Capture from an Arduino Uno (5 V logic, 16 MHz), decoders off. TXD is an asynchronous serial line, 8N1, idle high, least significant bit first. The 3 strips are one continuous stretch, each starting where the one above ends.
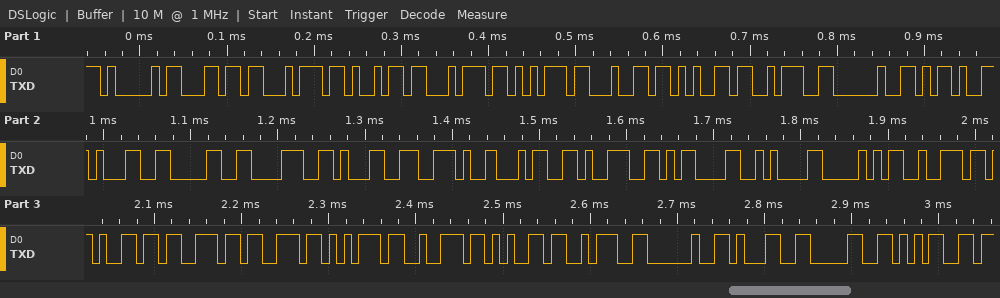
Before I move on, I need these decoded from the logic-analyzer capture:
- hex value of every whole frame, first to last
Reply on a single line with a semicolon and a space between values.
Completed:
41 6C 74 69 74 75 64 65 3A 20 2D 31 30 38 31 2E 34 39 0D 0A 50 72 65 73 73 75 72 65 3A 20 31 30 35
